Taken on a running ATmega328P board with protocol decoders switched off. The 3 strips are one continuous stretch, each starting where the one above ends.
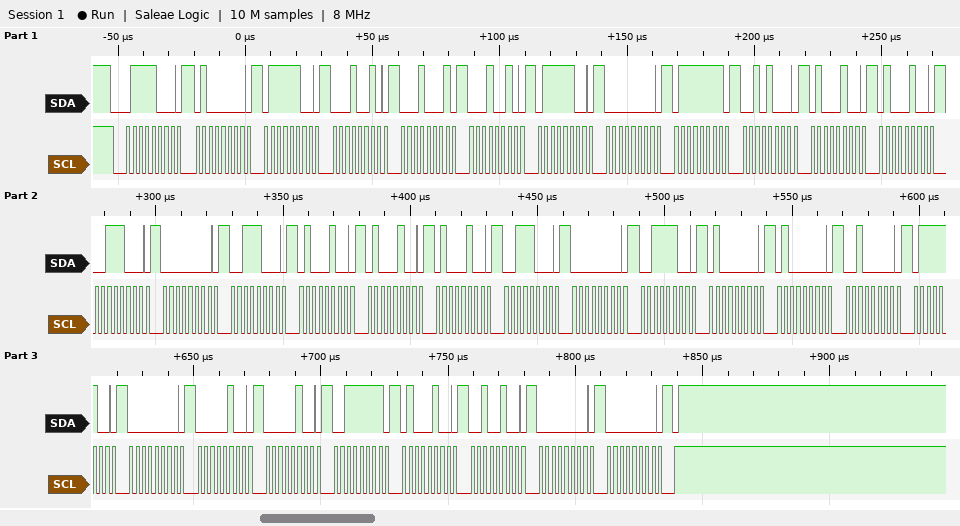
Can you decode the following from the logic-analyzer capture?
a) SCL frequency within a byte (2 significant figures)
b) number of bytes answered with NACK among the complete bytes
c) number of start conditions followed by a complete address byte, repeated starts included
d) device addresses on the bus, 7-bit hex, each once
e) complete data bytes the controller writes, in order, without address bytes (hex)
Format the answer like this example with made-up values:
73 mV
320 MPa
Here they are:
400 kHz
0
1
0x3C
40 7C 12 11 12 7C 00 7F 28 44 44 38 00 38 44 44 44 38 00 3C 40 40 20 7C 00 04 04 3F 44 24 00 00
